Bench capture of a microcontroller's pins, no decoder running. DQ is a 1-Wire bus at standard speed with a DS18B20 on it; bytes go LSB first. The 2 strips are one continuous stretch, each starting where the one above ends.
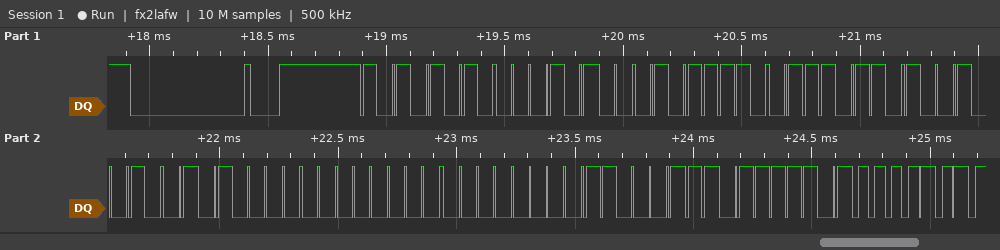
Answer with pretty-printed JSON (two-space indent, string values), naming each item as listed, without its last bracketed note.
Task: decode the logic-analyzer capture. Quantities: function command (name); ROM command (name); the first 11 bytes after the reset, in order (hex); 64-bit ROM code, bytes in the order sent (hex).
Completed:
{
  "function command": "Read Scratchpad",
  "ROM command": "Match ROM",
  "the first 11 bytes after the reset, in order": "55 28 7A 6E 49 0A 00 00 E3 BE 50",
  "64-bit ROM code, bytes in the order sent": "28 7A 6E 49 0A 00 00 E3"
}
